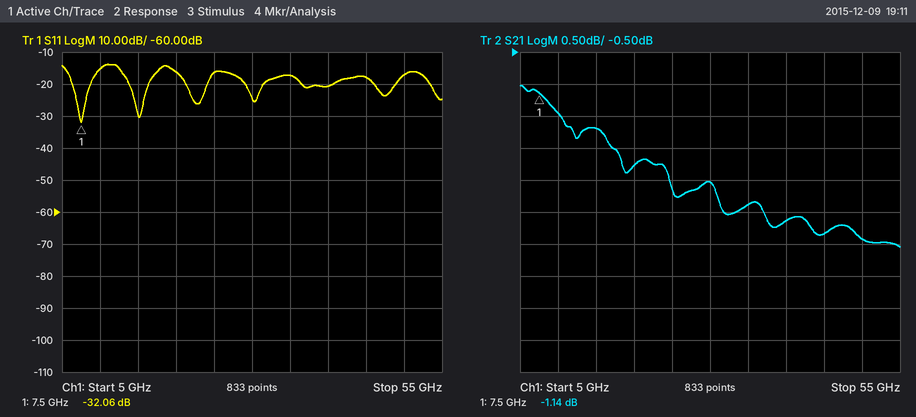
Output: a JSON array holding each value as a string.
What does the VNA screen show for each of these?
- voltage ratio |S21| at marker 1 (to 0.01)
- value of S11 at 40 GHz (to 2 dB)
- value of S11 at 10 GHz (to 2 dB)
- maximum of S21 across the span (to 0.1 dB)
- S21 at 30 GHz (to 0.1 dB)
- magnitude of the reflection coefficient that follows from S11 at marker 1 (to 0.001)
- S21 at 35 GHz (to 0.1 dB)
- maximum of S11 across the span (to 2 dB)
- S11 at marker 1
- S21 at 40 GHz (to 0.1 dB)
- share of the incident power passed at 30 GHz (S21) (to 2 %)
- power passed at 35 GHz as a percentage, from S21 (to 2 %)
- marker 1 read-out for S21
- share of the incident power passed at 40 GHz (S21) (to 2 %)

["0.88", "-20 dB", "-16 dB", "-1.0 dB", "-2.5 dB", "0.025", "-2.9 dB", "-14 dB", "-32.06 dB", "-3.1 dB", "56 %", "52 %", "-1.14 dB", "48 %"]
